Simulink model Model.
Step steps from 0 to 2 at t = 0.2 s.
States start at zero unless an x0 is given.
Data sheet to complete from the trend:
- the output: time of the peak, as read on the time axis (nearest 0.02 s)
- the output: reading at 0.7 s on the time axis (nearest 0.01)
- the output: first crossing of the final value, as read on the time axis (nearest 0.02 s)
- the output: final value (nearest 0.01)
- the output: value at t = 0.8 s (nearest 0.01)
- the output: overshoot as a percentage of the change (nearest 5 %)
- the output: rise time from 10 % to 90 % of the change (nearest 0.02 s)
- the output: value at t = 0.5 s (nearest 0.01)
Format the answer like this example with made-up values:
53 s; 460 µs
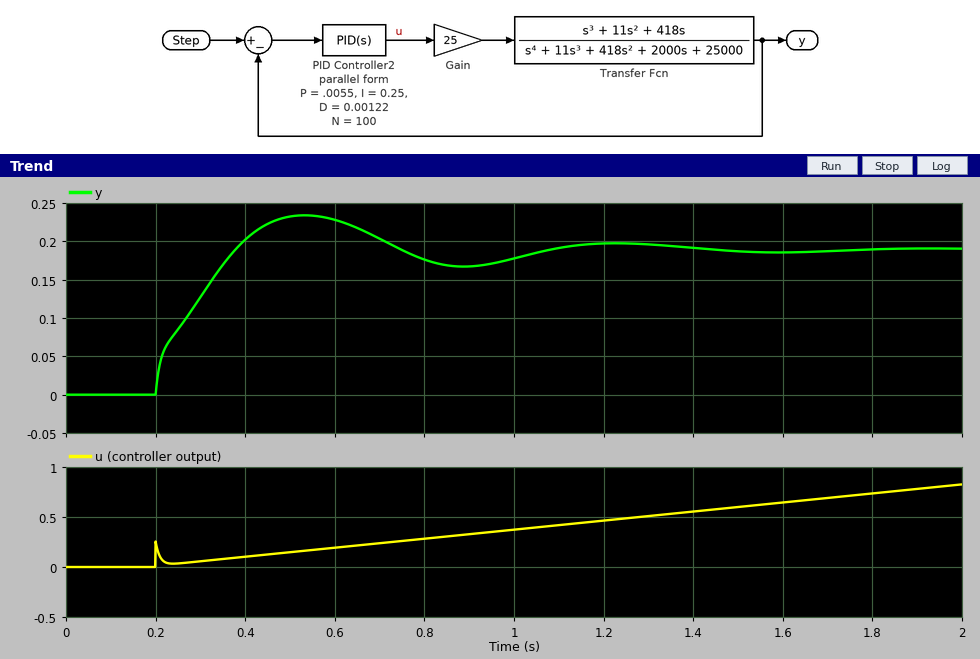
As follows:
0.54 s; 0.20; 0.38 s; 0.19; 0.18; 25 %; 0.14 s; 0.23
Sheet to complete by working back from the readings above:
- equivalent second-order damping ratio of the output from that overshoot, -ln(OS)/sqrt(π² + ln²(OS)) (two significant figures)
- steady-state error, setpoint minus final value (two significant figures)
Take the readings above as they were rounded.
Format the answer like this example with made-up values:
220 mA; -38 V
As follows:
0.40; 1.8
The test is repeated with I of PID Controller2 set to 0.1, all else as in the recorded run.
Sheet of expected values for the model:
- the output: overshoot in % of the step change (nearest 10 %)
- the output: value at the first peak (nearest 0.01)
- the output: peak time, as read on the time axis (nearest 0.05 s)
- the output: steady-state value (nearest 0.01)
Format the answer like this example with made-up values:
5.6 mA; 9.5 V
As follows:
20 %; 0.10; 0.35 s; 0.08
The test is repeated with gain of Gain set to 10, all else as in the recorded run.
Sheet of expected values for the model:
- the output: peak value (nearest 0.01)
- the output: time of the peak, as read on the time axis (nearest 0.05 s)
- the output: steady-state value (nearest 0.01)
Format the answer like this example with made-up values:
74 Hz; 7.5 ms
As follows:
0.10; 0.55 s; 0.08
